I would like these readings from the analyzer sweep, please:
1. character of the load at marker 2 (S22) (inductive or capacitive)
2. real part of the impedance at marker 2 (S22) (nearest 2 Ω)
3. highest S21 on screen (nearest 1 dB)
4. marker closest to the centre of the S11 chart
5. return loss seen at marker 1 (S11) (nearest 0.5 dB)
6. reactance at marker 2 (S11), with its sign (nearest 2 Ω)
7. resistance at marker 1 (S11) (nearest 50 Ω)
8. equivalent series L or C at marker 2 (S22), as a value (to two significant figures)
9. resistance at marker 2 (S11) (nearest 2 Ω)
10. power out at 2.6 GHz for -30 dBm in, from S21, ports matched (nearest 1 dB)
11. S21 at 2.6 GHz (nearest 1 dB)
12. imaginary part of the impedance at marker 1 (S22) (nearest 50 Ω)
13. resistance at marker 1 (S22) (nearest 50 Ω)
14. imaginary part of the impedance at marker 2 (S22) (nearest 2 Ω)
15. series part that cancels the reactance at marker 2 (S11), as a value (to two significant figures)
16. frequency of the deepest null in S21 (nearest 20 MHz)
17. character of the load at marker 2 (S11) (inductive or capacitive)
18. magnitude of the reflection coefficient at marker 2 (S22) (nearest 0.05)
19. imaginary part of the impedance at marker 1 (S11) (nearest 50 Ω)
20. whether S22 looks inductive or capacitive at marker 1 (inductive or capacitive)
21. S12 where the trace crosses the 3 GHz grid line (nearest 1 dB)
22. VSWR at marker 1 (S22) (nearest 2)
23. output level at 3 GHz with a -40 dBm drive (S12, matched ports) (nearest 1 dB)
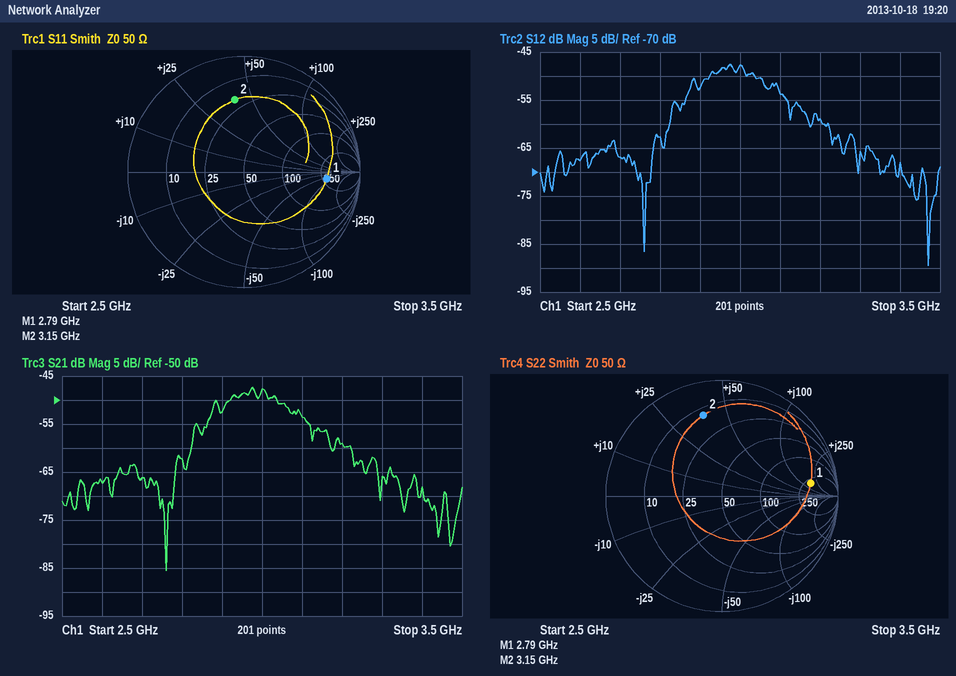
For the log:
inductive
14 Ω
-47 dB
marker 2
3.0 dB
+40 Ω
300 Ω
1.9 nH
20 Ω
-97 dBm
-67 dB
+150 Ω
300 Ω
+38 Ω
1.3 pF
2.76 GHz
inductive
0.70
-50 Ω
inductive
-48 dB
8
-88 dBm
